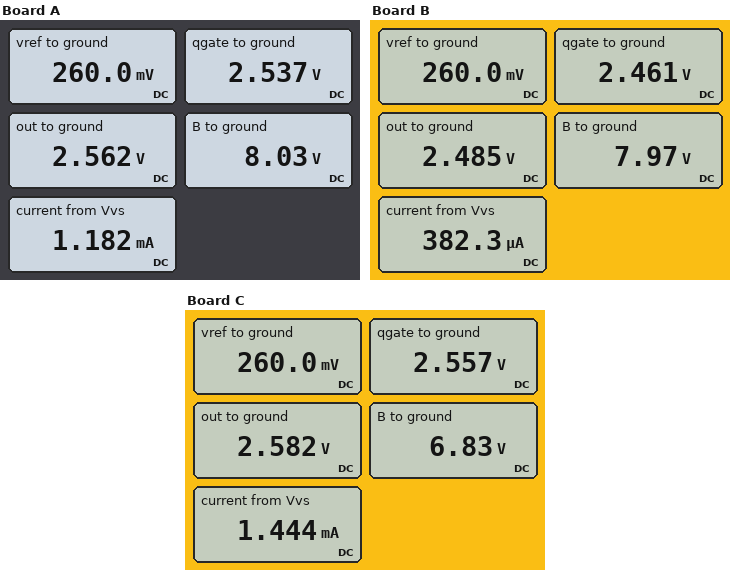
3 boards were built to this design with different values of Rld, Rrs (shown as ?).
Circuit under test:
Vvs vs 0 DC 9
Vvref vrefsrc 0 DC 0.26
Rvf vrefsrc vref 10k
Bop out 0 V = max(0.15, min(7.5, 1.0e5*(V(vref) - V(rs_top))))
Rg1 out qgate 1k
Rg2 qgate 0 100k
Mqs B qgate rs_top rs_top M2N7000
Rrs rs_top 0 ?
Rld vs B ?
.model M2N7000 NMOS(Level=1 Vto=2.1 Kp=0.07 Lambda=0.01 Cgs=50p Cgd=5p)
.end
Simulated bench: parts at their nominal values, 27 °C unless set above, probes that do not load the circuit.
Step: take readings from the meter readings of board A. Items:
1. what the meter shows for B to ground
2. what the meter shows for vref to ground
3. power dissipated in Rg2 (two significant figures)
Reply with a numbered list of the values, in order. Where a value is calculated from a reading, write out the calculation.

1. 8.03 V
2. 260.0 mV
3. (2.537 V)^2 / 100 kΩ = 64 µW
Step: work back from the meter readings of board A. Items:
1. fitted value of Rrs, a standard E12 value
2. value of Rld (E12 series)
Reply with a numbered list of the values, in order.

1. 220 Ω
2. 820 Ω
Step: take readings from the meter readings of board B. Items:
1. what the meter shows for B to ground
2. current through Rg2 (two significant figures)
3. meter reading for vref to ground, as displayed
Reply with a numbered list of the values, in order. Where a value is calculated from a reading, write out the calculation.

1. 7.97 V
2. (2.461 V) / 100 kΩ = 25 µA
3. 260.0 mV
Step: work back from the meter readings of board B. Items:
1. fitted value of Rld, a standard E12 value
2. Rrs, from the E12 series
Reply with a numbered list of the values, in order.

1. 2.7 kΩ
2. 680 Ω
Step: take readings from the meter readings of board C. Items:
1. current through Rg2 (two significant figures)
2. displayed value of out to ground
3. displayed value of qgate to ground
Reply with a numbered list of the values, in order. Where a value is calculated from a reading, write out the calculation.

1. (2.557 V) / 100 kΩ = 26 µA
2. 2.582 V
3. 2.557 V
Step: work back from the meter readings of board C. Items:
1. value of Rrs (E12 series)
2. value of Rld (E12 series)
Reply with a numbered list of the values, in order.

1. 180 Ω
2. 1.5 kΩ
